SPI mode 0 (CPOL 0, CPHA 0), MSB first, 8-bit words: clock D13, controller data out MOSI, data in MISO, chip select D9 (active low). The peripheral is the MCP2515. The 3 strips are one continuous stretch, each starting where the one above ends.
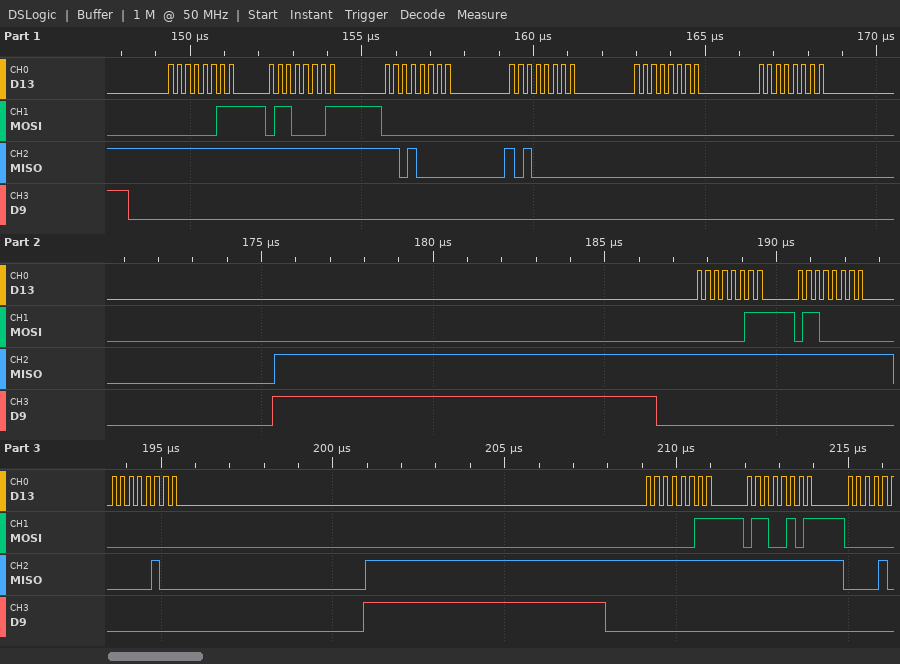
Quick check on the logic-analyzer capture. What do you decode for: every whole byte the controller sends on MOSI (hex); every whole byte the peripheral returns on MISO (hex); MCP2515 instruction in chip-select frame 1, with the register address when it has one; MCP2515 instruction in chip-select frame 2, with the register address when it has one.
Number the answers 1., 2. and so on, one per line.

1. 03 61 00 00 00 00 03 60 00 03 65
2. FF FF D0 A0 00 00 FF FF 04 FF FF
3. READ 0x61
4. READ 0x60
